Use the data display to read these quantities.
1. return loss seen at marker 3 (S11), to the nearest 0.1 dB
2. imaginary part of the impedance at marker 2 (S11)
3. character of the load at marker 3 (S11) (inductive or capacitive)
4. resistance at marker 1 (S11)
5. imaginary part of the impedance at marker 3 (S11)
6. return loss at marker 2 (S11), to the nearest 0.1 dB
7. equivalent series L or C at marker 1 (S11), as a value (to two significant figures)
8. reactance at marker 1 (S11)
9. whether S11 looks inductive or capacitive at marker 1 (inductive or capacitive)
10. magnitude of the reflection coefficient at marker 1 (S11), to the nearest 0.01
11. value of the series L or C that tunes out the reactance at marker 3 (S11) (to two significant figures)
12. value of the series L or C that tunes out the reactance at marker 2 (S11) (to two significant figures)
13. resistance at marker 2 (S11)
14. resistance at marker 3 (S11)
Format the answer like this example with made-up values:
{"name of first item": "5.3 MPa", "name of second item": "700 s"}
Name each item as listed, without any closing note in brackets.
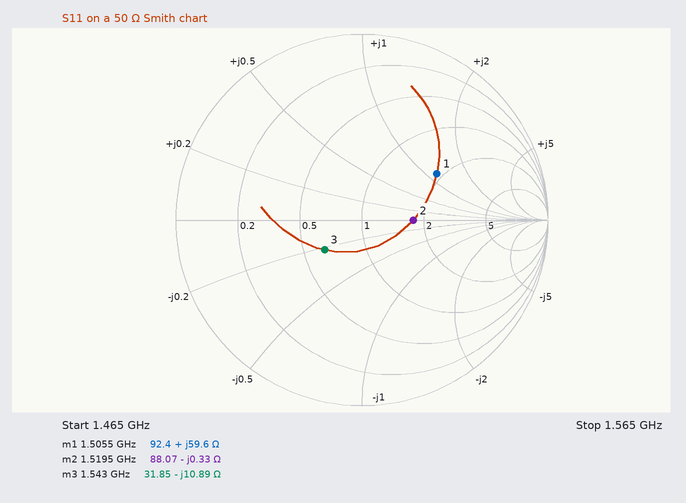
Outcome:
{"return loss seen at marker 3 (S11), to the nearest 0.1 dB": "11.8 dB", "imaginary part of the impedance at marker 2": "-0.33 Ω", "character of the load at marker 3 (S11)": "capacitive", "resistance at marker 1": "92.4 Ω", "imaginary part of the impedance at marker 3": "-10.89 Ω", "return loss at marker 2 (S11), to the nearest 0.1 dB": "11.2 dB", "equivalent series L or C at marker 1 (S11), as a value": "6.3 nH", "reactance at marker 1": "+59.6 Ω", "whether S11 looks inductive or capacitive at marker 1": "inductive", "magnitude of the reflection coefficient at marker 1 (S11), to the nearest 0.01": "0.47", "value of the series L or C that tunes out the reactance at marker 3 (S11)": "1.1 nH", "value of the series L or C that tunes out the reactance at marker 2 (S11)": "35 pH", "resistance at marker 2": "88.07 Ω", "resistance at marker 3": "31.85 Ω"}
